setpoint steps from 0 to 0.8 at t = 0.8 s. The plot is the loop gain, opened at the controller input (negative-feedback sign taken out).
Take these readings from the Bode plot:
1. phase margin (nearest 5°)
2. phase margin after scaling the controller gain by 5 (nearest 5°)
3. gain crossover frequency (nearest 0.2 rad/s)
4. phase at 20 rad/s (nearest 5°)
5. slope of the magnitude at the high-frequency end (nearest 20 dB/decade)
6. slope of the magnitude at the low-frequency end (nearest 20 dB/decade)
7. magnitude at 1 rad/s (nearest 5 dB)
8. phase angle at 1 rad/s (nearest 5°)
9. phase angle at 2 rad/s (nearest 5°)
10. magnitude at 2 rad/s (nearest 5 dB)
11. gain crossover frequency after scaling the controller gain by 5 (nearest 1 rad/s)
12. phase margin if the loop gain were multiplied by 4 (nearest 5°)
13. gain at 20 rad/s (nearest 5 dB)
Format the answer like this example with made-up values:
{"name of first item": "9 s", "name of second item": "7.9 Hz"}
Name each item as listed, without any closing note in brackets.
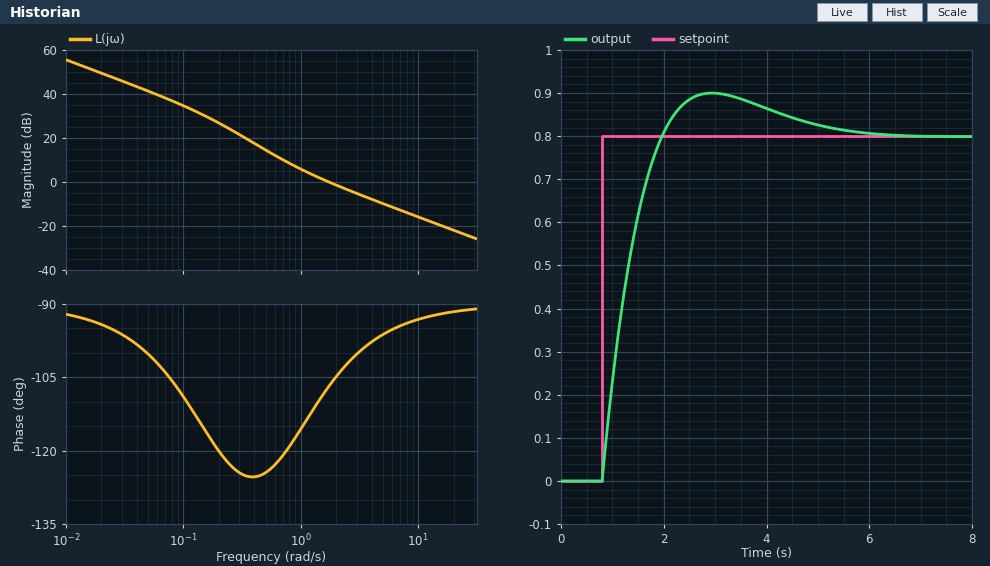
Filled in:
{"phase margin": "75°", "phase margin after scaling the controller gain by 5": "85°", "gain crossover frequency": "1.8 rad/s", "phase at 20 rad/s": "-90°", "slope of the magnitude at the high-frequency end": "-20 dB/decade", "slope of the magnitude at the low-frequency end": "-20 dB/decade", "magnitude at 1 rad/s": "5 dB", "phase angle at 1 rad/s": "-115°", "phase angle at 2 rad/s": "-105°", "magnitude at 2 rad/s": "0 dB", "gain crossover frequency after scaling the controller gain by 5": "8 rad/s", "phase margin if the loop gain were multiplied by 4": "85°", "gain at 20 rad/s": "-20 dB"}
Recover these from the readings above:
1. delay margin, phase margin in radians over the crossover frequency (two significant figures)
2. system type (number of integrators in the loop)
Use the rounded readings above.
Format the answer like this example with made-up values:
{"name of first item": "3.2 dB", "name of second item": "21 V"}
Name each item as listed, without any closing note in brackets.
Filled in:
{"delay margin, phase margin in radians over the crossover frequency": "0.73 s", "system type": "1"}
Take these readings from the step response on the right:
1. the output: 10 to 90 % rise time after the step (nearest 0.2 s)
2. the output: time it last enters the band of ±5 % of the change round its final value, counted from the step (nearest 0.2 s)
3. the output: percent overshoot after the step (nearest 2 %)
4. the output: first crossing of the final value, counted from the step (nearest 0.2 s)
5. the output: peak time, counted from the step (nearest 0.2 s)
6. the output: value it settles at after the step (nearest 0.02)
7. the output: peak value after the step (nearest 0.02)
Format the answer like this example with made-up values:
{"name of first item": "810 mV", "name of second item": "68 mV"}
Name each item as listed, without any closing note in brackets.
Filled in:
{"the output: 10 to 90 % rise time after the step": "0.8 s", "the output: time it last enters the band of ±5 % of the change round its final value, counted from the step": "3.8 s", "the output: percent overshoot after the step": "12 %", "the output: first crossing of the final value, counted from the step": "1.2 s", "the output: peak time, counted from the step": "2.2 s", "the output: value it settles at after the step": "0.80", "the output: peak value after the step": "0.90"}
